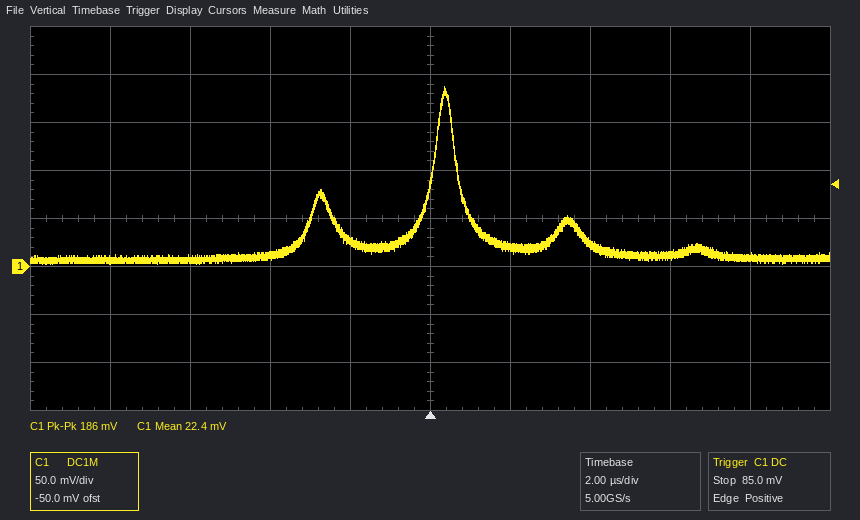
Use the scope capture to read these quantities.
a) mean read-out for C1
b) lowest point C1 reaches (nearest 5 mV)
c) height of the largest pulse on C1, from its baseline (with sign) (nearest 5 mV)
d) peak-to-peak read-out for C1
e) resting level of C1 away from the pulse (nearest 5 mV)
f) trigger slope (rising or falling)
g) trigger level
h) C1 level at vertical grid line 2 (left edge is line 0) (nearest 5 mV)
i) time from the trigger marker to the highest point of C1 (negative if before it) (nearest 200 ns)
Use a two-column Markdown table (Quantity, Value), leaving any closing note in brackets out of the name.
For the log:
| Quantity | Value |
|---|---|
| mean read-out for C1 | 22.4 mV |
| lowest point C1 reaches | 0 mV |
| height of the largest pulse on C1, from its baseline (with sign) | +180 mV |
| peak-to-peak read-out for C1 | 186 mV |
| resting level of C1 away from the pulse | 10 mV |
| trigger slope | rising |
| trigger level | 85.0 mV |
| C1 level at vertical grid line 2 (left edge is line 0) | 10 mV |
| time from the trigger marker to the highest point of C1 (negative if before it) | +400 ns |
